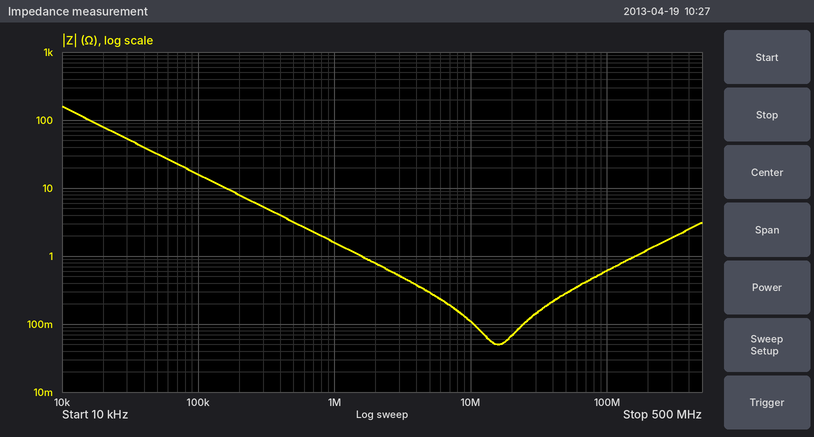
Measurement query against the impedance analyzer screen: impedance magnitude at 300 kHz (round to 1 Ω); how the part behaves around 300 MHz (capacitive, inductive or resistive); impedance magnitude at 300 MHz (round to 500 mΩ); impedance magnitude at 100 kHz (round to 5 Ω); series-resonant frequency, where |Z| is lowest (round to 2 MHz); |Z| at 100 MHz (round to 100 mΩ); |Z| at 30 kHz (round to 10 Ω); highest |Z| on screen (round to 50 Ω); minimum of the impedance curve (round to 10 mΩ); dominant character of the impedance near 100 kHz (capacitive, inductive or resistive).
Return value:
5 Ω
inductive
2.0 Ω
15 Ω
16 MHz
600 mΩ
50 Ω
150 Ω
50 mΩ
capacitive
